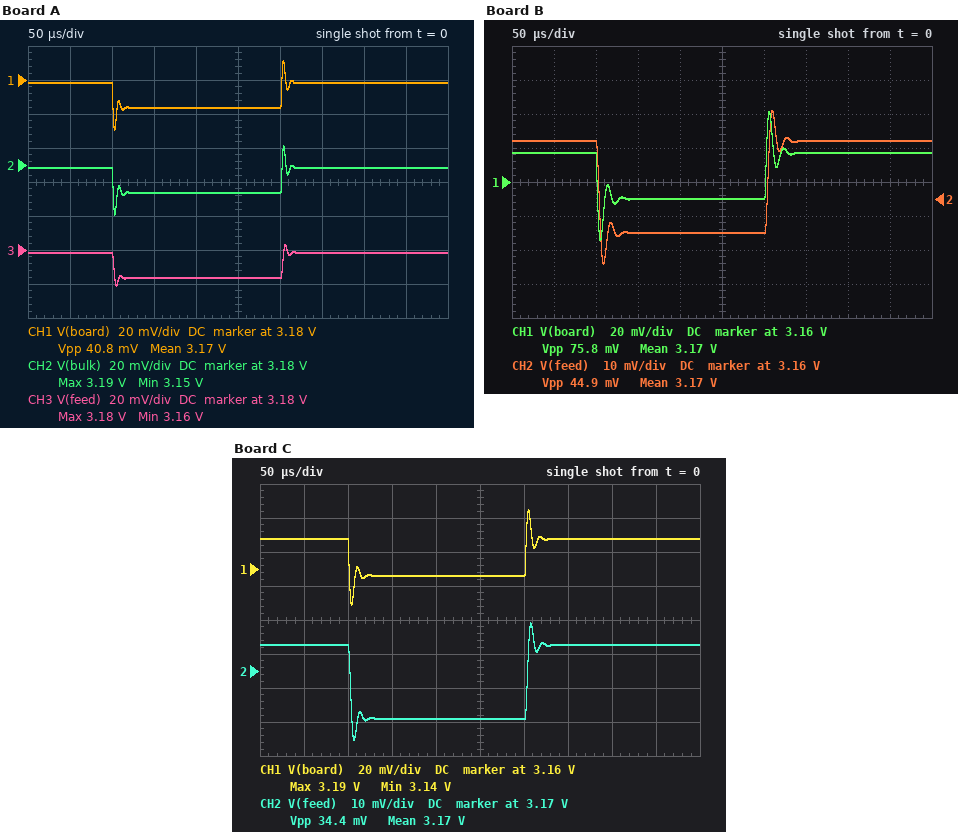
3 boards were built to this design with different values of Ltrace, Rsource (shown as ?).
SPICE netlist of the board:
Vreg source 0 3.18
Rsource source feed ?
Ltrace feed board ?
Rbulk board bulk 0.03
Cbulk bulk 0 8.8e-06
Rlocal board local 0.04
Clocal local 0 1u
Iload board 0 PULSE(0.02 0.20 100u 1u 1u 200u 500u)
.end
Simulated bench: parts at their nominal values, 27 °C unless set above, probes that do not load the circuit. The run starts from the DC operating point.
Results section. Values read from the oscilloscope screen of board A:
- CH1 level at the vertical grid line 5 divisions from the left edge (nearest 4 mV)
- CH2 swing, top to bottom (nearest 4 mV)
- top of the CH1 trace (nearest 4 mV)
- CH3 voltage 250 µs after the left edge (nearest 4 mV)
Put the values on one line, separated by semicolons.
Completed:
3.164 V; 40 mV; 3.192 V; 3.164 V
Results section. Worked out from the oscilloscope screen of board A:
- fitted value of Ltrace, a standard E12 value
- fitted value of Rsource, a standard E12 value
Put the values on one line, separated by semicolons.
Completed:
220 nH; 0.082 Ω
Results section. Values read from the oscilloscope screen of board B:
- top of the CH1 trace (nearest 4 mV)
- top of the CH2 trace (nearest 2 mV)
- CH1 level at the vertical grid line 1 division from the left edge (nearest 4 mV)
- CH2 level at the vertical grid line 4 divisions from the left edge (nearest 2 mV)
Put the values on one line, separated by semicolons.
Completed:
3.200 V; 3.186 V; 3.176 V; 3.150 V
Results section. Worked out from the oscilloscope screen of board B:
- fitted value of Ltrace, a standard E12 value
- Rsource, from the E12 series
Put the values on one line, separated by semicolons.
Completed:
680 nH; 0.15 Ω
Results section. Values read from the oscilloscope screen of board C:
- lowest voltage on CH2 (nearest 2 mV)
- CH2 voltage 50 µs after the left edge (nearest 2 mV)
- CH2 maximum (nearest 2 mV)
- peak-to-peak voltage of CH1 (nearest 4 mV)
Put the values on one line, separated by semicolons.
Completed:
3.150 V; 3.178 V; 3.184 V; 56 mV
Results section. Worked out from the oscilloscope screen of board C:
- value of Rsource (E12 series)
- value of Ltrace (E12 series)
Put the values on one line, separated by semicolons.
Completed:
0.12 Ω; 390 nH
